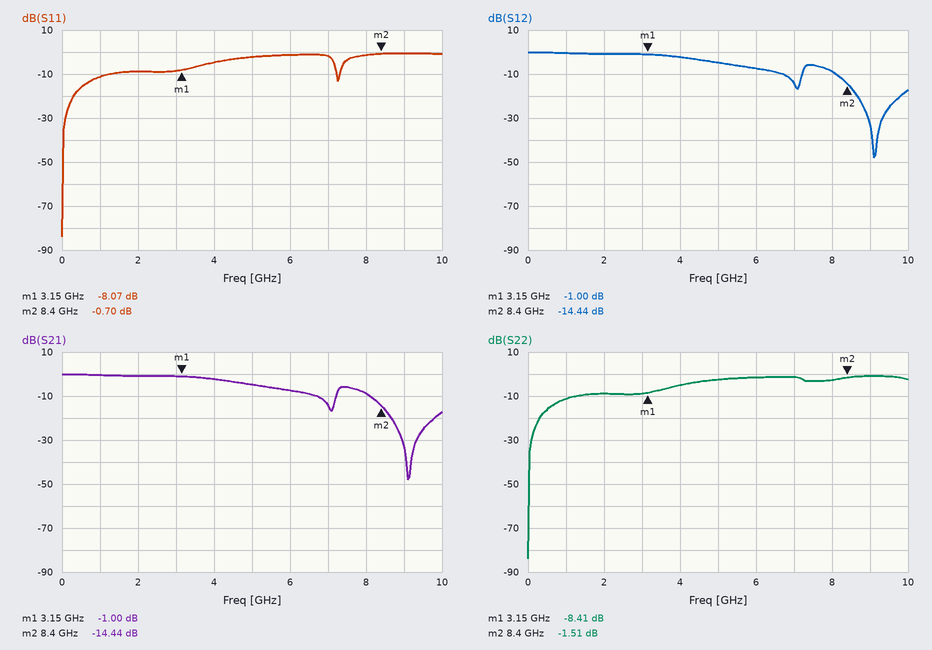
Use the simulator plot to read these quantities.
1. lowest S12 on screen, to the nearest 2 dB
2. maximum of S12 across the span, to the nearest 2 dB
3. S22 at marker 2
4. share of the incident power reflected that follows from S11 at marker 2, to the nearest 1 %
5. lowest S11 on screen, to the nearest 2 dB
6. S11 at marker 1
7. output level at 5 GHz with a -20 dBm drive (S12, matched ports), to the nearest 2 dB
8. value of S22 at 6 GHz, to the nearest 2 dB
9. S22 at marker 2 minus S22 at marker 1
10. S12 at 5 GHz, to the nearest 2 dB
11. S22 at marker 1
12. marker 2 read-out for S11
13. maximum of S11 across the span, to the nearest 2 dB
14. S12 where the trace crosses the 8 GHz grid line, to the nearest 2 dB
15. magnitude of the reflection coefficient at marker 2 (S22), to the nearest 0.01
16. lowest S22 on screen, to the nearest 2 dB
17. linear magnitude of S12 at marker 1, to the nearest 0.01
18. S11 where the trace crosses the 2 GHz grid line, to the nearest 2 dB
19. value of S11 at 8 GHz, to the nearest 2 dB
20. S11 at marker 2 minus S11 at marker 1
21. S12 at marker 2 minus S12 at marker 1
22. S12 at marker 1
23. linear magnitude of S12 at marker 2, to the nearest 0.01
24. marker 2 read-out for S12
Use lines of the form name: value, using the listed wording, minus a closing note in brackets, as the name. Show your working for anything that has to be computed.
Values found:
lowest S12 on screen, to the nearest 2 dB: -48 dB
maximum of S12 across the span, to the nearest 2 dB: 0 dB
S22 at marker 2: -1.51 dB
share of the incident power reflected that follows from S11 at marker 2, to the nearest 1 %: 10^(-0.7/10) ≈ 85 %
lowest S11 on screen, to the nearest 2 dB: -84 dB
S11 at marker 1: -8.07 dB
output level at 5 GHz with a -20 dBm drive (S12, matched ports), to the nearest 2 dB: -20 dBm + (-4 dB) = -24 dBm
value of S22 at 6 GHz, to the nearest 2 dB: -2 dB
S22 at marker 2 minus S22 at marker 1: -1.51 − (-8.41) = 6.90 dB
S12 at 5 GHz, to the nearest 2 dB: -4 dB
S22 at marker 1: -8.41 dB
marker 2 read-out for S11: -0.70 dB
maximum of S11 across the span, to the nearest 2 dB: 0 dB
S12 where the trace crosses the 8 GHz grid line, to the nearest 2 dB: -8 dB
magnitude of the reflection coefficient at marker 2 (S22), to the nearest 0.01: 10^(-1.51/20) ≈ 0.84
lowest S22 on screen, to the nearest 2 dB: -84 dB
linear magnitude of S12 at marker 1, to the nearest 0.01: 10^(-1/20) ≈ 0.89
S11 where the trace crosses the 2 GHz grid line, to the nearest 2 dB: -8 dB
value of S11 at 8 GHz, to the nearest 2 dB: -2 dB
S11 at marker 2 minus S11 at marker 1: -0.7 − (-8.07) = 7.37 dB
S12 at marker 2 minus S12 at marker 1: -14.44 − (-1) = -13.44 dB
S12 at marker 1: -1.00 dB
linear magnitude of S12 at marker 2, to the nearest 0.01: 10^(-14.44/20) ≈ 0.19
marker 2 read-out for S12: -14.44 dB
